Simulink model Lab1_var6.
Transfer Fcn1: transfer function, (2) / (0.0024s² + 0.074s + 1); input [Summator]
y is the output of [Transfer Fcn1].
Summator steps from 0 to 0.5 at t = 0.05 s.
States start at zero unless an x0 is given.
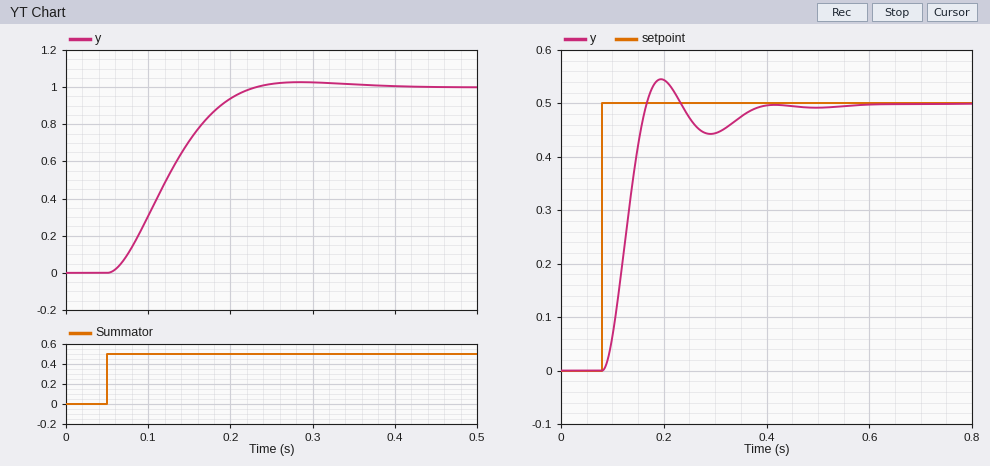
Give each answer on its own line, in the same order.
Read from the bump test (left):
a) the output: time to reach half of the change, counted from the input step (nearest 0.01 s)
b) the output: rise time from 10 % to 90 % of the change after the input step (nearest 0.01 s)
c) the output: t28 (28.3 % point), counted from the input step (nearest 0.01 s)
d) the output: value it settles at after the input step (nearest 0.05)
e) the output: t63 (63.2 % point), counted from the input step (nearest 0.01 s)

0.07 s
0.11 s
0.05 s
1.00
0.09 s
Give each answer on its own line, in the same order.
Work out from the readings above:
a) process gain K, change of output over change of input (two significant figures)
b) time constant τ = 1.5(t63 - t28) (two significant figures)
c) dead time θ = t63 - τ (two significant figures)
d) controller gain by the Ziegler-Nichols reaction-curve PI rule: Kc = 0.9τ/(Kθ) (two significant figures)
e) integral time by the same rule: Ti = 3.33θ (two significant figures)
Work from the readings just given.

2.0
0.060 s
0.030 s
0.90
0.100 s
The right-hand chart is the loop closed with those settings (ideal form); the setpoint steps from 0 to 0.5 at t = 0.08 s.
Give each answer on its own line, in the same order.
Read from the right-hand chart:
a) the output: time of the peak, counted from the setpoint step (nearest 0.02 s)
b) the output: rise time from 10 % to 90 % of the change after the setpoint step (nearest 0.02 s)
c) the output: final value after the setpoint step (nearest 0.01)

0.12 s
0.06 s
0.50
